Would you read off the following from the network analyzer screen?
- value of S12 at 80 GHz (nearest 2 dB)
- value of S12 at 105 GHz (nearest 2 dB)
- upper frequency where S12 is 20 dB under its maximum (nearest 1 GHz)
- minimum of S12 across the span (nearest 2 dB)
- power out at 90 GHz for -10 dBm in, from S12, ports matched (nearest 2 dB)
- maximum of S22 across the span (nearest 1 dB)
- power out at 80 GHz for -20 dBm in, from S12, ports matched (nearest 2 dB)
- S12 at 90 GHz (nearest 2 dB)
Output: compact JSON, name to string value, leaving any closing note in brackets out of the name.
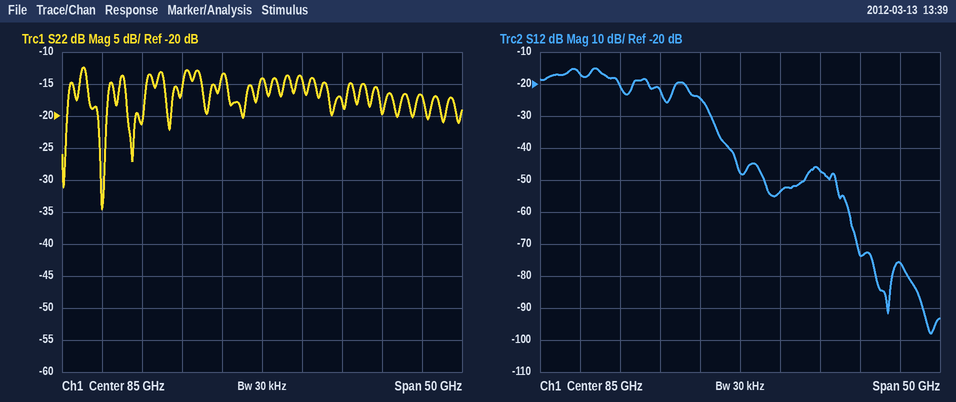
{"value of S12 at 80 GHz": "-24 dB", "value of S12 at 105 GHz": "-76 dB", "upper frequency where S12 is 20 dB under its maximum": "82 GHz", "minimum of S12 across the span": "-98 dB", "power out at 90 GHz for -10 dBm in, from S12, ports matched": "-64 dBm", "maximum of S22 across the span": "-12 dB", "power out at 80 GHz for -20 dBm in, from S12, ports matched": "-44 dBm", "S12 at 90 GHz": "-54 dB"}
